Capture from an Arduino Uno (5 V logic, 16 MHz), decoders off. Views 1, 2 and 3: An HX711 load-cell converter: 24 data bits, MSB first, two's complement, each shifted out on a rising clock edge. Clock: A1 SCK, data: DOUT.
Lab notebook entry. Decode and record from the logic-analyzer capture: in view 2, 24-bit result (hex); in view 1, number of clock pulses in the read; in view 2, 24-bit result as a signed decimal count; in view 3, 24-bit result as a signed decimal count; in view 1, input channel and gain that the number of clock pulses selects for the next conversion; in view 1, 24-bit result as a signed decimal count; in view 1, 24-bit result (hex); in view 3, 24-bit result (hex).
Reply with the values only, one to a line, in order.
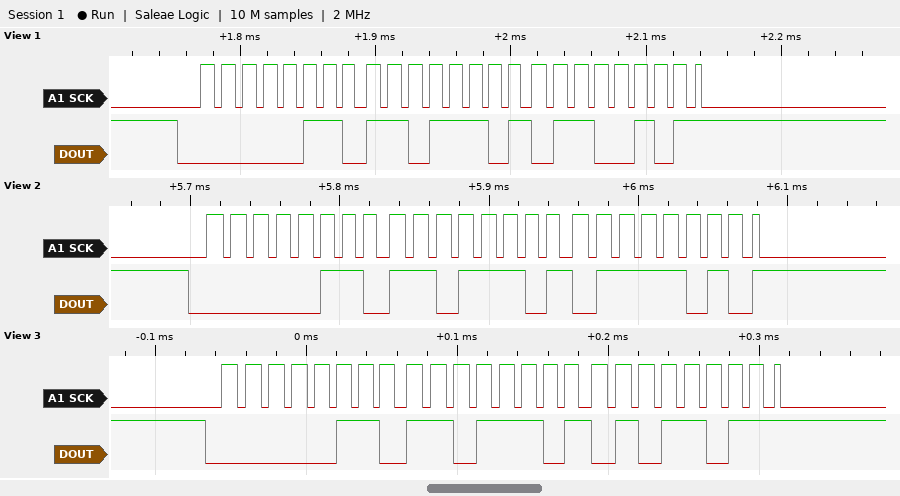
0x06DD7A
25
449914
449883
channel A, gain 128
449893
0x06DD65
0x06DD5B
